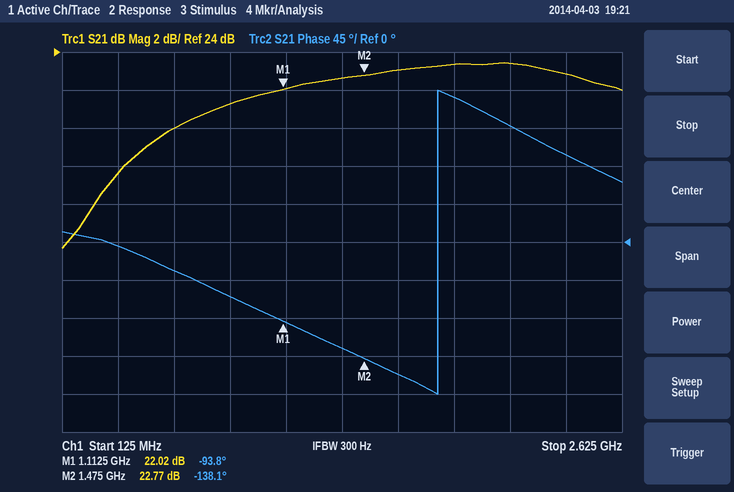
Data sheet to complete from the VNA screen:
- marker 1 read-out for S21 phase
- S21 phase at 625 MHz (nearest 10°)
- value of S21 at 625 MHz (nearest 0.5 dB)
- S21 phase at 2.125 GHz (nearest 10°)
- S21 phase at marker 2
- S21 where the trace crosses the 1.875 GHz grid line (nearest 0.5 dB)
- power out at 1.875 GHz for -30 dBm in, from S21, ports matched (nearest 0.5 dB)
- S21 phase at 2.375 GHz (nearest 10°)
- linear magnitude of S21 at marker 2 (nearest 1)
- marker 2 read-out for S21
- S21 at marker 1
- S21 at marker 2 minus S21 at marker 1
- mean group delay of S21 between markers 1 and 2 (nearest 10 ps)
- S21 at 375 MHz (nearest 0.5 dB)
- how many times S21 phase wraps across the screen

-93.8°
-30°
20.0 dB
140°
-138.1°
23.5 dB
-6.5 dBm
100°
14
22.77 dB
22.02 dB
0.75 dB
340 ps
17.5 dB
1
